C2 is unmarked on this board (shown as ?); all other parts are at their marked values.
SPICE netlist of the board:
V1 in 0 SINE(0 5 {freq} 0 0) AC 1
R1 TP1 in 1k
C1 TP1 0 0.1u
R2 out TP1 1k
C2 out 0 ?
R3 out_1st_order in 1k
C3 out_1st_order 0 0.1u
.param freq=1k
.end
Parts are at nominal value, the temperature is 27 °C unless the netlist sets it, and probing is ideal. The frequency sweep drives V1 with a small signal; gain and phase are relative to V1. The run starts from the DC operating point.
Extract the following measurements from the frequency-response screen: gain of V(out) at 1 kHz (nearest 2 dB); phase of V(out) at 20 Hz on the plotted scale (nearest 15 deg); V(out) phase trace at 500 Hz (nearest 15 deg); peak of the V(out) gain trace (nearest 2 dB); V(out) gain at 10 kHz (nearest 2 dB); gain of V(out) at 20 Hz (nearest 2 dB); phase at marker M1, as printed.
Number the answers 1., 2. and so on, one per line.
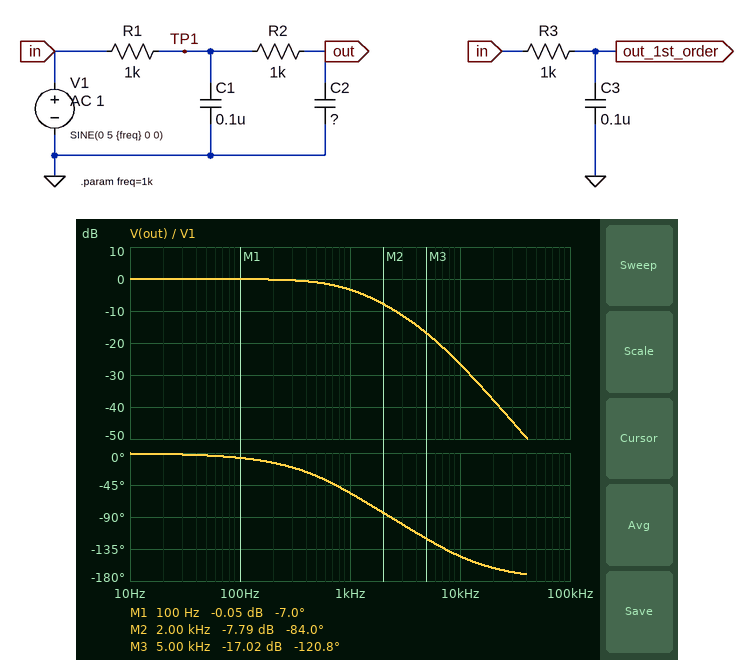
1. -4 dB
2. 0 deg
3. -30 deg
4. 0 dB
5. -26 dB
6. 0 dB
7. -7.0 deg
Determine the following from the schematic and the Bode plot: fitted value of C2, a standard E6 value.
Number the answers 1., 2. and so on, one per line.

1. 47 nF
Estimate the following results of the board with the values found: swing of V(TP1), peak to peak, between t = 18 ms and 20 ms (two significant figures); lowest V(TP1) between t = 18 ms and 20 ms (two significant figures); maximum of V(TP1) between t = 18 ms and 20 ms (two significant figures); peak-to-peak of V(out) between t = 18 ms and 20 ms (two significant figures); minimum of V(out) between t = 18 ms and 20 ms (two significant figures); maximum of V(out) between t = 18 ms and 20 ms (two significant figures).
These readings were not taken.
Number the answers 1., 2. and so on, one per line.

1. 7.1 V
2. -3.6 V
3. 3.6 V
4. 6.8 V
5. -3.4 V
6. 3.4 V
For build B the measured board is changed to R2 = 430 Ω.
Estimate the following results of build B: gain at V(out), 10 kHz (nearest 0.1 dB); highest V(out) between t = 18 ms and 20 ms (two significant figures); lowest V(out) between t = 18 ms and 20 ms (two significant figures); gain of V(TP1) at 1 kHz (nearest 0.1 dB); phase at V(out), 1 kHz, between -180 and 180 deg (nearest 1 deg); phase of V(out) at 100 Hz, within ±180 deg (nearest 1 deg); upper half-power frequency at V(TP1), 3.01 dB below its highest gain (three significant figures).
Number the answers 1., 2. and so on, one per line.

1. -22.0 dB
2. 3.6 V
3. -3.6 V
4. -2.8 dB
5. -49 deg
6. -6 deg
7. 1.04 kHz
